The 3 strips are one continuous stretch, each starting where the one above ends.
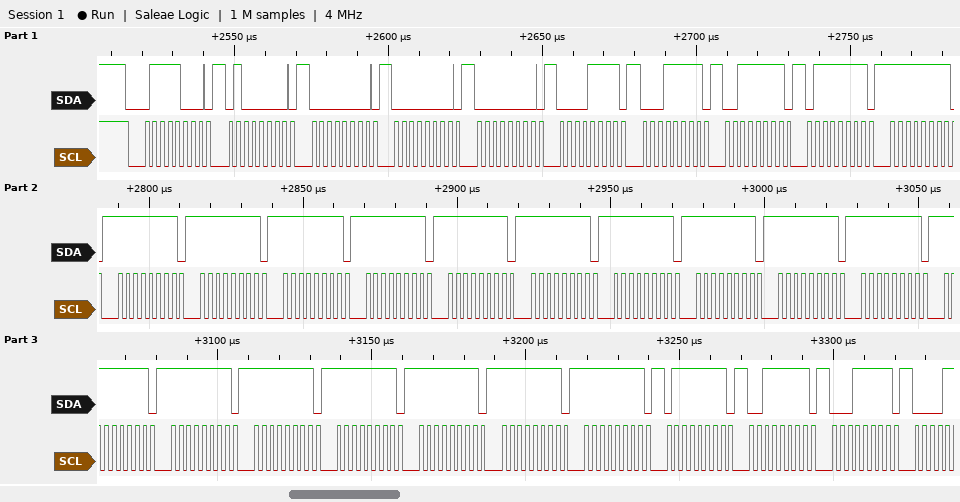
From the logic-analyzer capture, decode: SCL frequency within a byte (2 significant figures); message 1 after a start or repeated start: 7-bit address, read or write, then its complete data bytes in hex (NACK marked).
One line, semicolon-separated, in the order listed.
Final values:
400 kHz; 0x3C write: 40 00 00 00 0F 1F 3F 7F FF FF FF FF FF FF FF FF FF FF FF FF FF FF FF FF FF FF 7F 3F 1F
